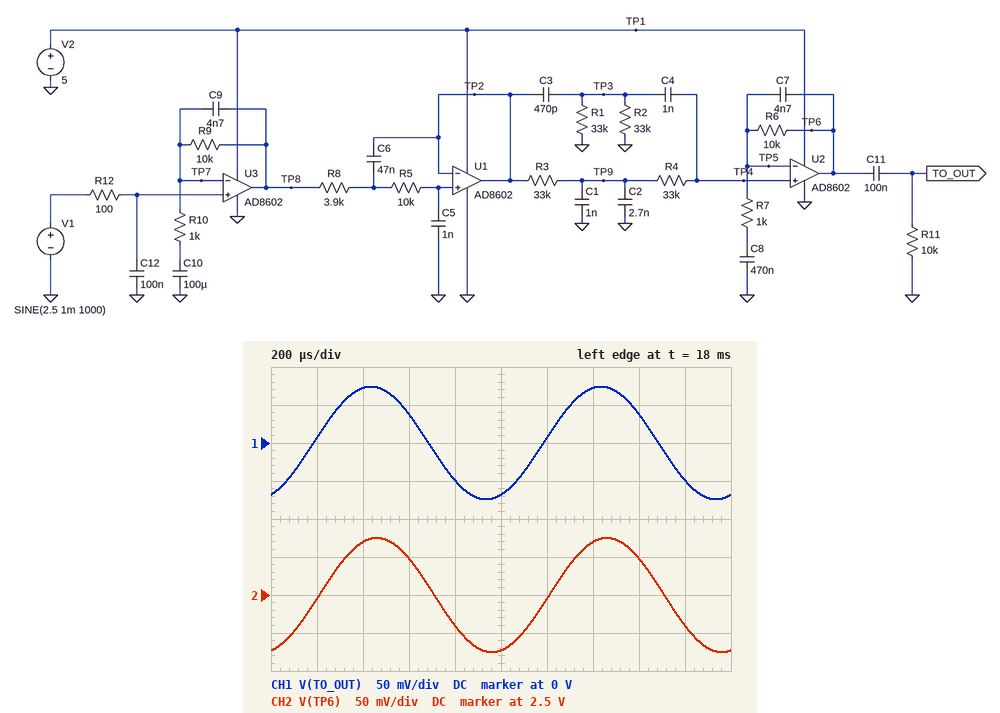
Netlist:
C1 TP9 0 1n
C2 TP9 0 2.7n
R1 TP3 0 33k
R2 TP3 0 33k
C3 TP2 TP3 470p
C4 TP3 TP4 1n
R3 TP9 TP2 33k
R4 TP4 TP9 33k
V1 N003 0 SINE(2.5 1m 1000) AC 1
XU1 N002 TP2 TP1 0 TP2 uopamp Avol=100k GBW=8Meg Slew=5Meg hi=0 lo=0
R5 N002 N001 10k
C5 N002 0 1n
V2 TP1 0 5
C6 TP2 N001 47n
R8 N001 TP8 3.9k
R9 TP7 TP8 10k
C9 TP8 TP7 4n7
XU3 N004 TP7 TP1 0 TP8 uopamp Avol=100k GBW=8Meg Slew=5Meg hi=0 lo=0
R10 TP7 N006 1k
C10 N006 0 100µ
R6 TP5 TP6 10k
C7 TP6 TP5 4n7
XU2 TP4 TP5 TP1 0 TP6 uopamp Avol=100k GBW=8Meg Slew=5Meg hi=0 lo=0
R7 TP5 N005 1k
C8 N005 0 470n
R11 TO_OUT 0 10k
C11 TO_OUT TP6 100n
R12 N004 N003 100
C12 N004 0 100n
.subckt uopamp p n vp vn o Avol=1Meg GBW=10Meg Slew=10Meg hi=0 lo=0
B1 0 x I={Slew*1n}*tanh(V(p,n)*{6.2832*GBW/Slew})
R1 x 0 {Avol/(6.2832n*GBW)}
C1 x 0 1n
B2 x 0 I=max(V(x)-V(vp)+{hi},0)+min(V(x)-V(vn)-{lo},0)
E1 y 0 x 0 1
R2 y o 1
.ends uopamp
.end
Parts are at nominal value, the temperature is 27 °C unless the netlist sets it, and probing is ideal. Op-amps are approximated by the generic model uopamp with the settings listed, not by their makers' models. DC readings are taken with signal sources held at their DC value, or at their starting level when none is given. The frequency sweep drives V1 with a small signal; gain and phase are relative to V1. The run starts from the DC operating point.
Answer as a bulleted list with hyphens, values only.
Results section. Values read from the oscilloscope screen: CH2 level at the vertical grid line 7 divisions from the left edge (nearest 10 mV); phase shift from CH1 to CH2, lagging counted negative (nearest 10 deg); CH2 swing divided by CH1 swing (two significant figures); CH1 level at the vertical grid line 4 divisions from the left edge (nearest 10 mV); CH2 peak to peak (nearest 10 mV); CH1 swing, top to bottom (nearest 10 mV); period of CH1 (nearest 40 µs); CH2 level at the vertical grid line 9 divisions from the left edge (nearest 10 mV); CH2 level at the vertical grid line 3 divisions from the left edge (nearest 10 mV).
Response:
- 2.57 V
- -10 deg
- 1.0
- -50 mV
- 150 mV
- 150 mV
- 1.00 ms
- 2.46 V
- 2.55 V
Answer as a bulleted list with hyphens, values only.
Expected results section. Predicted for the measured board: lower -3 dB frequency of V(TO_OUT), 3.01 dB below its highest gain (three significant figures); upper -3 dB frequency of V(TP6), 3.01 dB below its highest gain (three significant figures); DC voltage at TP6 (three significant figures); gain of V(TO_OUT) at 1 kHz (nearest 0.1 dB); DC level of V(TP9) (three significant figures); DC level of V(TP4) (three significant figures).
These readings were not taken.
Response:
- 254 Hz
- 1.34 kHz
- 2.50 V
- 37.4 dB
- 2.50 V
- 2.50 V
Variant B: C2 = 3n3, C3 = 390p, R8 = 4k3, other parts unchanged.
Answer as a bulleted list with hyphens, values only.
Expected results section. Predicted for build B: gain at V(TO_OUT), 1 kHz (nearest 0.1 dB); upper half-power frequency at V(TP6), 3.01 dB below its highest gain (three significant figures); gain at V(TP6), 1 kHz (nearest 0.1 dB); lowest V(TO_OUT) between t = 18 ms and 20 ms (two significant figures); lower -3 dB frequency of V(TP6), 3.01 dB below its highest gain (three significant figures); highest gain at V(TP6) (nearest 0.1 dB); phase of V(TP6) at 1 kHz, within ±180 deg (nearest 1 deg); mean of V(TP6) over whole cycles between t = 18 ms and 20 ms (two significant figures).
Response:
- 37.0 dB
- 1.28 kHz
- 37.1 dB
- -71 mV
- 200 Hz
- 38.7 dB
- -79 deg
- 2.5 V
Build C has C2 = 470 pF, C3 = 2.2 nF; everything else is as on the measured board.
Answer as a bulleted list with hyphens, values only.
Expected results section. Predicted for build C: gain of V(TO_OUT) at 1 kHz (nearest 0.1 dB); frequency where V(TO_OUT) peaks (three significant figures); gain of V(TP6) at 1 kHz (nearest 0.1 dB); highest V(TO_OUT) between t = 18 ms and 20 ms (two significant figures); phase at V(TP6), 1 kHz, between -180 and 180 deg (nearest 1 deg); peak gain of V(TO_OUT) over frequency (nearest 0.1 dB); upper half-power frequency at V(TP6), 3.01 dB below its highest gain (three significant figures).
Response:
- 38.6 dB
- 659 Hz
- 38.7 dB
- 85 mV
- -57 deg
- 39.2 dB
- 1.50 kHz
